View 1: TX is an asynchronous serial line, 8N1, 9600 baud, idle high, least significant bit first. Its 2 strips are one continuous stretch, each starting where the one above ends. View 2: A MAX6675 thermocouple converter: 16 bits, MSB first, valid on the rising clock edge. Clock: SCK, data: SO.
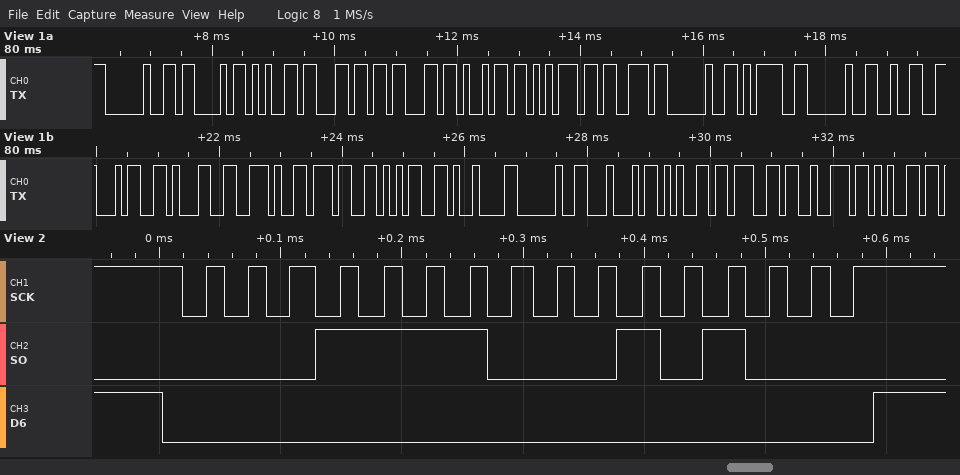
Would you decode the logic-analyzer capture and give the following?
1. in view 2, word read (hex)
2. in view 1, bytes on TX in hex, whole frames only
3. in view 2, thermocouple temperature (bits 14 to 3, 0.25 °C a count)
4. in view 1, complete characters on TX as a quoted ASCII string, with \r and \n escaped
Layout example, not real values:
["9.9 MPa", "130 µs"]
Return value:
["0x1E28", "20 43 65 6C 63 69 75 73 20 3D 20 32 34 31 2E 37 35 09 20 44 65 67 72 65", "241.25 °C", "\" Celcius = 241.75\\t Degre\""]
